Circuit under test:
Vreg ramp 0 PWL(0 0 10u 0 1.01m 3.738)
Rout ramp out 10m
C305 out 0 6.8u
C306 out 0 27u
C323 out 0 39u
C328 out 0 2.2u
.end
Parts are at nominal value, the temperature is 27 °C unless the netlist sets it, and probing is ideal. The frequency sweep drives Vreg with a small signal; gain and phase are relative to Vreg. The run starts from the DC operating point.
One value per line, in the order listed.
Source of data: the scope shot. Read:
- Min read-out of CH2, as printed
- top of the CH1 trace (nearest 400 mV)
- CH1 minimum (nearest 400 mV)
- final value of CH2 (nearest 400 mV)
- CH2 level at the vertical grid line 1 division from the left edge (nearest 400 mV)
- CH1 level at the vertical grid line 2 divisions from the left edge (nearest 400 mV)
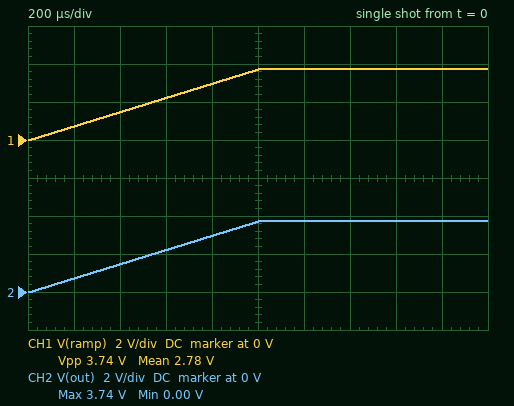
0.00 V
3.6 V
0 V
3.6 V
800 mV
1.6 V
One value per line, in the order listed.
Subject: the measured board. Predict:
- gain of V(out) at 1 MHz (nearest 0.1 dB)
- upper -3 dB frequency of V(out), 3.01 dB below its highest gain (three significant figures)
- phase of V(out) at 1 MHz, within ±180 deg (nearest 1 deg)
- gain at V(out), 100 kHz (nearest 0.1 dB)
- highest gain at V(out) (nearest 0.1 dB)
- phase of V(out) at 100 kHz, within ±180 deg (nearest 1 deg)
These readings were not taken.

-13.7 dB
212 kHz
-78 deg
-0.9 dB
0 dB
-25 deg
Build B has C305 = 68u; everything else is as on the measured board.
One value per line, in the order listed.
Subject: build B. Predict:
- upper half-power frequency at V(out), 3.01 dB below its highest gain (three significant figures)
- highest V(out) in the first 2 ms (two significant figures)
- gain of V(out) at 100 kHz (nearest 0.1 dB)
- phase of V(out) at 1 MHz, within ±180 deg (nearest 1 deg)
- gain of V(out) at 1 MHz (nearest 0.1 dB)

117 kHz
3.7 V
-2.4 dB
-83 deg
-18.7 dB
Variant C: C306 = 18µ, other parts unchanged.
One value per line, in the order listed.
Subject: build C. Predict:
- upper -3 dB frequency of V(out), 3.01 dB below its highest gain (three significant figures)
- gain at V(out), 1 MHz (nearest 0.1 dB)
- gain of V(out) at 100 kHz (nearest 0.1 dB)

241 kHz
-12.6 dB
-0.7 dB
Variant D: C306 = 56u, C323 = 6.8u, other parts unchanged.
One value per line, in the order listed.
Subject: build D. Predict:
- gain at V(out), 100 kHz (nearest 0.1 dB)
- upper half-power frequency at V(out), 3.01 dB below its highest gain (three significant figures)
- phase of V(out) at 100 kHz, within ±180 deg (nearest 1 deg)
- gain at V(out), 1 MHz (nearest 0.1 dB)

-0.8 dB
222 kHz
-24 deg
-13.3 dB
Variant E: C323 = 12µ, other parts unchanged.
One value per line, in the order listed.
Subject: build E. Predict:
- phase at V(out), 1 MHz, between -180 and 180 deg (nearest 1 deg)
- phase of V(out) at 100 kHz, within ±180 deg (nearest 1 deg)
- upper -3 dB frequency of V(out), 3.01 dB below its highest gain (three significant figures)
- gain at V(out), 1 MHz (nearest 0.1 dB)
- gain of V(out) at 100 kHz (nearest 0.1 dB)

-72 deg
-17 deg
332 kHz
-10.0 dB
-0.4 dB
